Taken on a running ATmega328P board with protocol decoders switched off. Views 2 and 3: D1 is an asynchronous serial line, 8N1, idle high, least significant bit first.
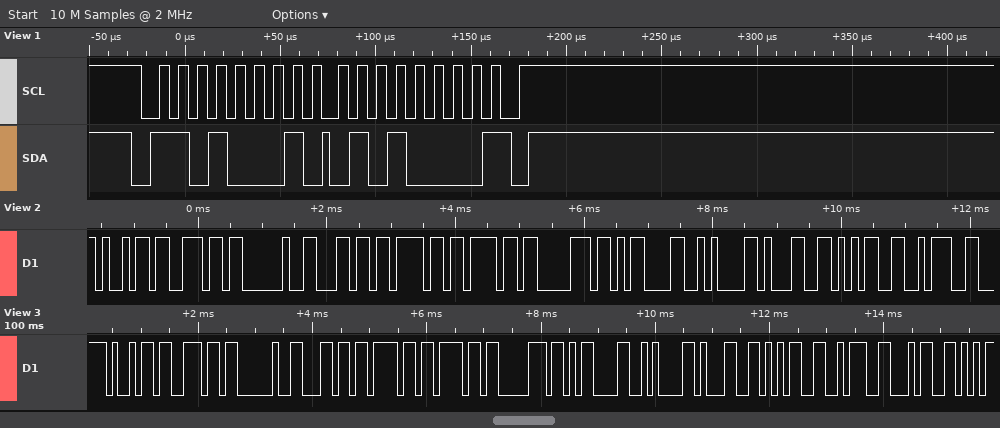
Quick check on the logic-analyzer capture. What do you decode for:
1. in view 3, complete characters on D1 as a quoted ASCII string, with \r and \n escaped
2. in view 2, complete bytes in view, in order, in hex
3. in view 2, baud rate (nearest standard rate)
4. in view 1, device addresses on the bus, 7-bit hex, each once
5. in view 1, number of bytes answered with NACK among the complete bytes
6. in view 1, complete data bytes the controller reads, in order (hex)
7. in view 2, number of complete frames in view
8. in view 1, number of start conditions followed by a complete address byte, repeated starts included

"in loop\r\n15:4"
69 6E 20 6C 6F 6F 70 0D 0A 31 35 3A
9600 baud
0x68
1
50
12
1
